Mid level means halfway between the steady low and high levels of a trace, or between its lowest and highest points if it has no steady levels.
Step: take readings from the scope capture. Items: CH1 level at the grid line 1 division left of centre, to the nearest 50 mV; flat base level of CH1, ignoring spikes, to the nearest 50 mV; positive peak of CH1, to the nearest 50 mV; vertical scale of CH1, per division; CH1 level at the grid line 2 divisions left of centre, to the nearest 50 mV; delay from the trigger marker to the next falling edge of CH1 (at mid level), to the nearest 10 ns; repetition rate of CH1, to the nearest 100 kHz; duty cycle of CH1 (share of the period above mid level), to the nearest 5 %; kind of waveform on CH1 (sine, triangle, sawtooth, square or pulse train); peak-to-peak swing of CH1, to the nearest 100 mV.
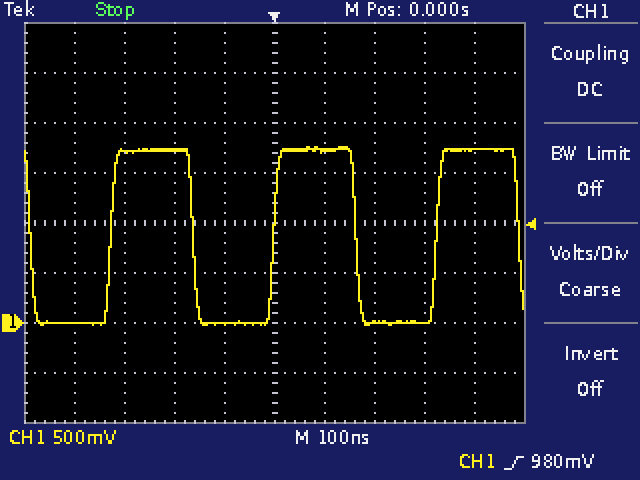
0 mV
0 mV
1.75 V
500 mV
1.75 V
160 ns
3.1 MHz
50 %
square
1.80 V
